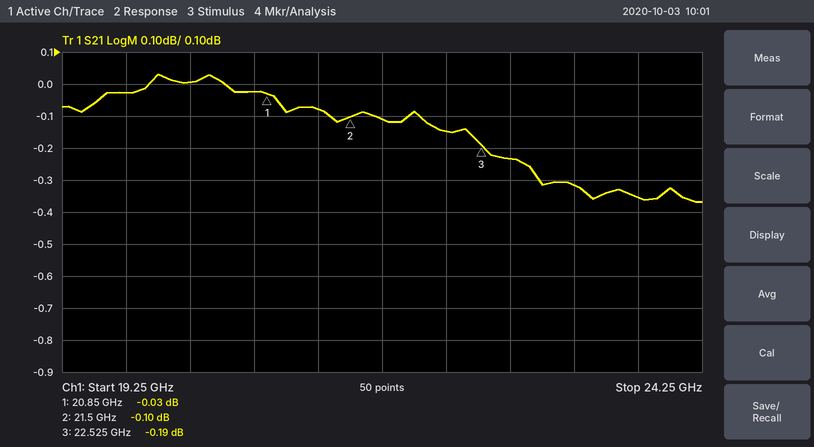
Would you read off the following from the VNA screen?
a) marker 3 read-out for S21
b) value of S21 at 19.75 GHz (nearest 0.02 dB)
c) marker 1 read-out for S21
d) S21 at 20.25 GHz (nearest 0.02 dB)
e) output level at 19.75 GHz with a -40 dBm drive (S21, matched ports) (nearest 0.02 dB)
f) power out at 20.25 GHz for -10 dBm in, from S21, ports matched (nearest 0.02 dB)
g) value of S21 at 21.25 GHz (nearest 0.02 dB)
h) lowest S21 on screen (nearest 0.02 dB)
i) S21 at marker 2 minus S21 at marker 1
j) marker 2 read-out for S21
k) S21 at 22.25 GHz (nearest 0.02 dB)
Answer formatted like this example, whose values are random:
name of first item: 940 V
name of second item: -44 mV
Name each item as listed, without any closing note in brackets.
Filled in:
marker 3 read-out for S21: -0.19 dB
value of S21 at 19.75 GHz: -0.02 dB
marker 1 read-out for S21: -0.03 dB
S21 at 20.25 GHz: 0.00 dB
output level at 19.75 GHz with a -40 dBm drive (S21, matched ports): -40.02 dBm
power out at 20.25 GHz for -10 dBm in, from S21, ports matched: -10.00 dBm
value of S21 at 21.25 GHz: -0.08 dB
lowest S21 on screen: -0.36 dB
S21 at marker 2 minus S21 at marker 1: -0.07 dB
marker 2 read-out for S21: -0.10 dB
S21 at 22.25 GHz: -0.14 dB
